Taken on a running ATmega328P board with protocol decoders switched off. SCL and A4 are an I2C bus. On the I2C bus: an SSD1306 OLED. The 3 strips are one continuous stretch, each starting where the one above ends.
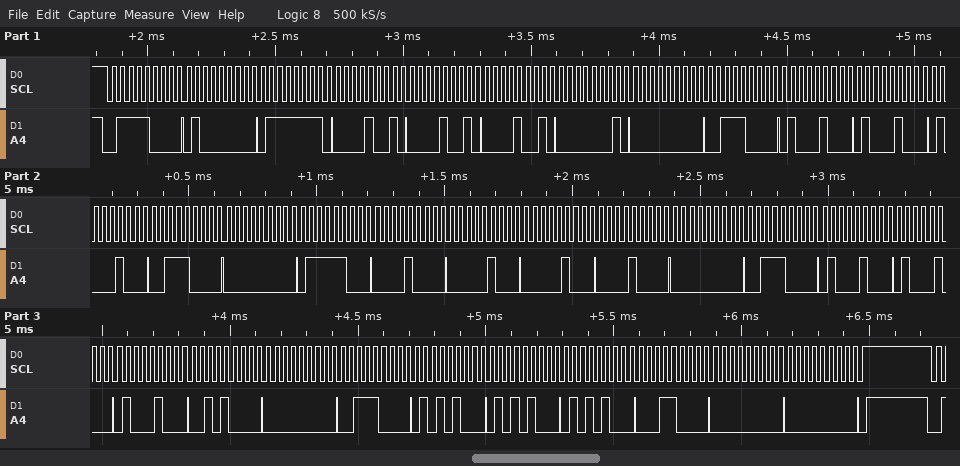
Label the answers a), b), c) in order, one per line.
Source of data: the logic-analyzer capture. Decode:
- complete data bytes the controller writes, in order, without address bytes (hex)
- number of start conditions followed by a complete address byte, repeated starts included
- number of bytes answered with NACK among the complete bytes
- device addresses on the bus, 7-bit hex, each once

a) 40 7F 09 09 09 01 00 38 44 44 44 38 00 7C 08 04 04 08 00 38 44 44 44 28 00 38 54 54 54 18 00 00
b) 1
c) 0
d) 0x3C
